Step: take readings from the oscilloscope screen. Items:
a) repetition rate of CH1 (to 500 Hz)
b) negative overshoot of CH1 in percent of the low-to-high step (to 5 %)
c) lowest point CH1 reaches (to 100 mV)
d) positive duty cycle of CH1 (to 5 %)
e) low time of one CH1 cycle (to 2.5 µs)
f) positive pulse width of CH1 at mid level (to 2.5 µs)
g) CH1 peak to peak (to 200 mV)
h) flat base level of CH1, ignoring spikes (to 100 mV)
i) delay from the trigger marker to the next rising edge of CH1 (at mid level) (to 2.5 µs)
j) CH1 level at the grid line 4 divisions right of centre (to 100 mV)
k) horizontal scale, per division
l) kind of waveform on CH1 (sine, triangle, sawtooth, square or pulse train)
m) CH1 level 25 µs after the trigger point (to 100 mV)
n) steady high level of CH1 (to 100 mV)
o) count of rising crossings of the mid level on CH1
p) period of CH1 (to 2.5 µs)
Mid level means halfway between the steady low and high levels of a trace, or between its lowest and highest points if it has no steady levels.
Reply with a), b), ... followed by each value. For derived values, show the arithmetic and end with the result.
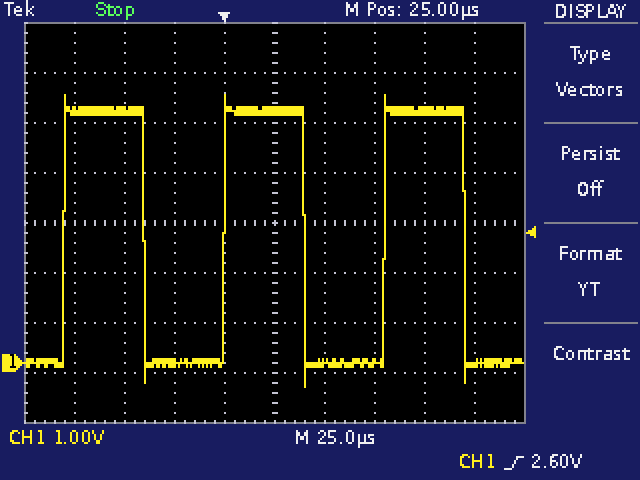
a) 1 / 80.0 µs ≈ 12.5 kHz
b) 10 %
c) -500 mV
d) 40.0 µs / 80.0 µs ≈ 50 %
e) 40.0 µs
f) 40.0 µs
g) 5.8 V
h) 0.0 V
i) 80.0 µs
j) 0.0 V
k) 25 µs
l) square
m) 5.0 V
n) 5.0 V
o) 3
p) 80.0 µs
